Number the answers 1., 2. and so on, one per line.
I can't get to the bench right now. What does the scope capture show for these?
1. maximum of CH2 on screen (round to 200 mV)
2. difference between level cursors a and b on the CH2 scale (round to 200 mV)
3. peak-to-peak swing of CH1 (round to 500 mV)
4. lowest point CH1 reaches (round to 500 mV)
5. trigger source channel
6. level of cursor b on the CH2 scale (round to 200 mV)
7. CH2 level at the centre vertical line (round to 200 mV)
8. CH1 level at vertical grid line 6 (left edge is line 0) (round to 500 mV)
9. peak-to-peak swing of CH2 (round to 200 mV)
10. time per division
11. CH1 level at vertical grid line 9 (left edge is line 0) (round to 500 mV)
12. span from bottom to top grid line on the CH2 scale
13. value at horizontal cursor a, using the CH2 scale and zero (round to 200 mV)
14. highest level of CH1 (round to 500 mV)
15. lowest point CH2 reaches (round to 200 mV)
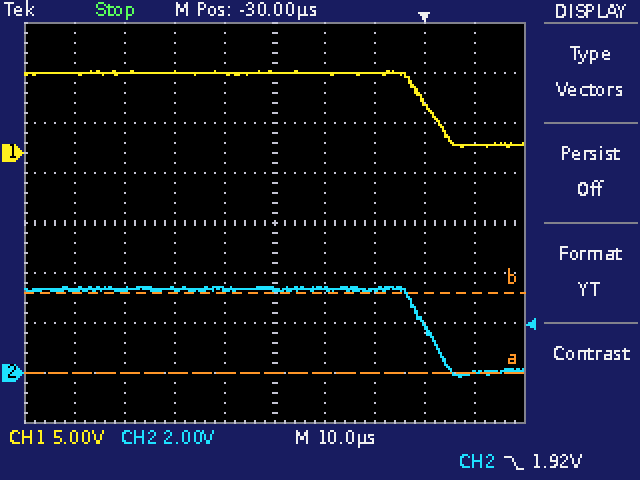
1. 3.4 V
2. 3.2 V
3. 7.5 V
4. 500 mV
5. CH2
6. 3.2 V
7. 3.4 V
8. 8.0 V
9. 3.6 V
10. 10 µs
11. 1.0 V
12. 16 V
13. 0.0 V
14. 8.0 V
15. -200 mV
